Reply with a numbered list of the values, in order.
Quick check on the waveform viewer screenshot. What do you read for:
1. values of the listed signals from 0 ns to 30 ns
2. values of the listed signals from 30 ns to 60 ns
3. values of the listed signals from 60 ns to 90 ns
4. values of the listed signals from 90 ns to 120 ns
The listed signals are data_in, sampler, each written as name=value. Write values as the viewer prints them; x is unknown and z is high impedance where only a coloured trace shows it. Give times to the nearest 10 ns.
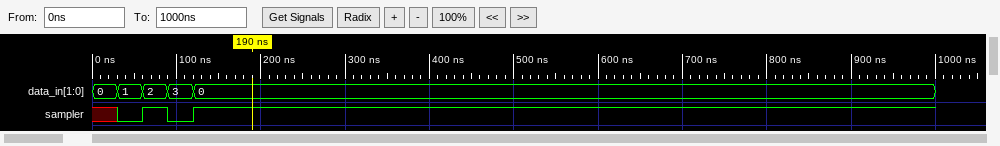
1. data_in=0, sampler=x
2. data_in=1, sampler=0
3. data_in=2, sampler=1
4. data_in=3, sampler=0
